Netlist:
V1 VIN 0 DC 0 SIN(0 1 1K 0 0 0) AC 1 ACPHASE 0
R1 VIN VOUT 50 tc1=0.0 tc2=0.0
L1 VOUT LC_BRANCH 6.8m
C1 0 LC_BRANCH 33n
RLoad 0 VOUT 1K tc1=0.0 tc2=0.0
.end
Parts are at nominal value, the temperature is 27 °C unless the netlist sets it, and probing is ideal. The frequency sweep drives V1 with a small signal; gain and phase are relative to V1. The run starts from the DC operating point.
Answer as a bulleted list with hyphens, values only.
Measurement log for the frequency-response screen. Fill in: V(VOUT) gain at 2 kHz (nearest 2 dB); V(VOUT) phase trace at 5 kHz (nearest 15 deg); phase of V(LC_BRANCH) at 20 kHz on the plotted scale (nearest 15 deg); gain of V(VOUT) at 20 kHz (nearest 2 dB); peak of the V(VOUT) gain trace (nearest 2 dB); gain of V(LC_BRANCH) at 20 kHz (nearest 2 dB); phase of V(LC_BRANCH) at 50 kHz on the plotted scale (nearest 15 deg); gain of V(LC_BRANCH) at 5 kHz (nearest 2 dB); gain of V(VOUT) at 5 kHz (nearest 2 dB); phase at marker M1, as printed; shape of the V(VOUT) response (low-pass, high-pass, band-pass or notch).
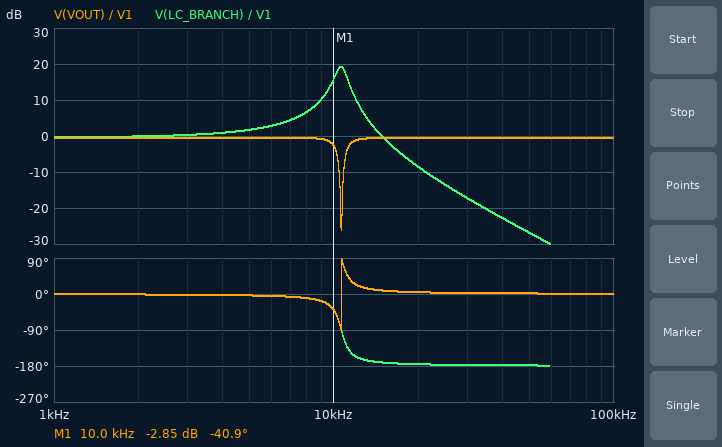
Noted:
- 0 dB
- 0 deg
- -180 deg
- 0 dB
- 0 dB
- -8 dB
- -180 deg
- 2 dB
- 0 dB
- -40.9 deg
- notch
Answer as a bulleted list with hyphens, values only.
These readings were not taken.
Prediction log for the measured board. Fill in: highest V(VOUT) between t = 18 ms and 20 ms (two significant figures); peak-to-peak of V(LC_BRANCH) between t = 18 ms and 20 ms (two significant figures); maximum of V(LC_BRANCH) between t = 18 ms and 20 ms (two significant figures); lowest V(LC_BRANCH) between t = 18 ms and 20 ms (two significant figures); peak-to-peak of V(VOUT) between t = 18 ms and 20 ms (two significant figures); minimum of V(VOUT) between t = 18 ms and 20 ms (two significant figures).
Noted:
- 950 mV
- 1.9 V
- 960 mV
- -960 mV
- 1.9 V
- -950 mV
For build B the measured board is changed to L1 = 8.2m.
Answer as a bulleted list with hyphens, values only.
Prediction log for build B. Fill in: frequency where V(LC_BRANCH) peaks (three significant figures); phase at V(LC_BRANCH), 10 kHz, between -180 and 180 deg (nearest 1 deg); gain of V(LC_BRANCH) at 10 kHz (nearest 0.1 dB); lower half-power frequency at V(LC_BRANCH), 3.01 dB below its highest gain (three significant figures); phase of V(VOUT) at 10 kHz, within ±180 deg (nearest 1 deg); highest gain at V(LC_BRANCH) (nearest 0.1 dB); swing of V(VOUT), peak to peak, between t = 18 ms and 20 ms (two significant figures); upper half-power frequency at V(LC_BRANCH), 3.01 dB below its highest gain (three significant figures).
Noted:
- 9.65 kHz
- -125 deg
- 18.0 dB
- 9.18 kHz
- 55 deg
- 20.0 dB
- 1.9 V
- 10.1 kHz
